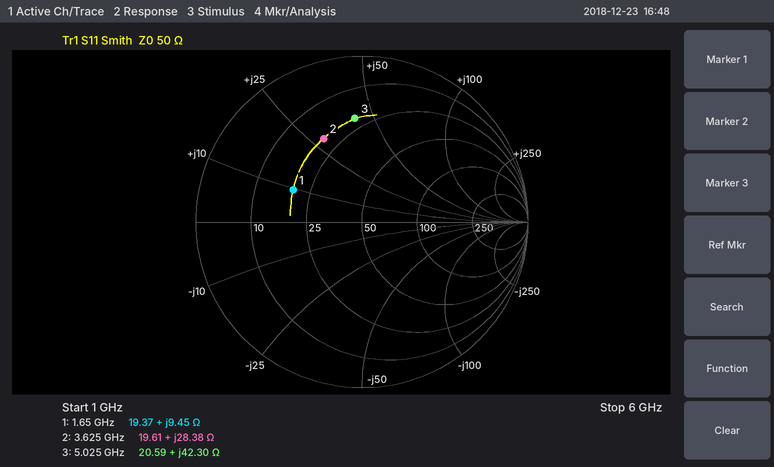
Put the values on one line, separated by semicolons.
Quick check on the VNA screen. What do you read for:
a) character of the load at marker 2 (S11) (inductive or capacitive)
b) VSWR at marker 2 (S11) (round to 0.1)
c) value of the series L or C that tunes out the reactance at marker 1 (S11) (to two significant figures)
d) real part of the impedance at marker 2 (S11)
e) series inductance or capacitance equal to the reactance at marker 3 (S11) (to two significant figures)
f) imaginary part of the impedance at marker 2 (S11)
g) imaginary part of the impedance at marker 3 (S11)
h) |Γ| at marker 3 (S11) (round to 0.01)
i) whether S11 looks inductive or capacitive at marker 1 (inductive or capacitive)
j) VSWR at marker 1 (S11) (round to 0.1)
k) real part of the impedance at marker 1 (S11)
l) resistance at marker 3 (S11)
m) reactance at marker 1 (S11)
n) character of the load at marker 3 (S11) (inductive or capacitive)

inductive; 3.5; 10 pF; 19.61 Ω; 1.3 nH; +28.38 Ω; +42.30 Ω; 0.63; inductive; 2.7; 19.37 Ω; 20.59 Ω; +9.45 Ω; inductive
